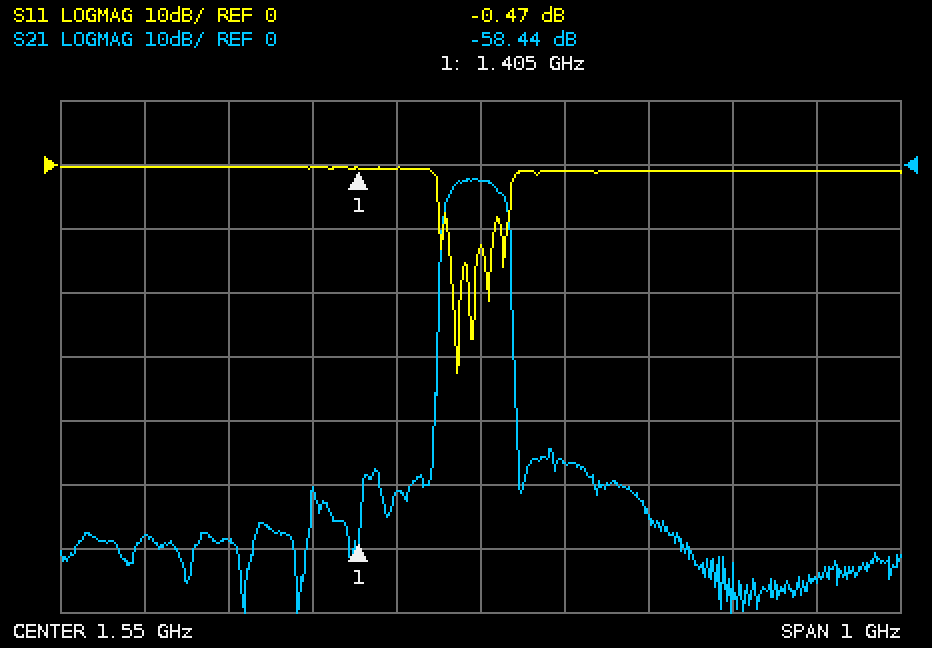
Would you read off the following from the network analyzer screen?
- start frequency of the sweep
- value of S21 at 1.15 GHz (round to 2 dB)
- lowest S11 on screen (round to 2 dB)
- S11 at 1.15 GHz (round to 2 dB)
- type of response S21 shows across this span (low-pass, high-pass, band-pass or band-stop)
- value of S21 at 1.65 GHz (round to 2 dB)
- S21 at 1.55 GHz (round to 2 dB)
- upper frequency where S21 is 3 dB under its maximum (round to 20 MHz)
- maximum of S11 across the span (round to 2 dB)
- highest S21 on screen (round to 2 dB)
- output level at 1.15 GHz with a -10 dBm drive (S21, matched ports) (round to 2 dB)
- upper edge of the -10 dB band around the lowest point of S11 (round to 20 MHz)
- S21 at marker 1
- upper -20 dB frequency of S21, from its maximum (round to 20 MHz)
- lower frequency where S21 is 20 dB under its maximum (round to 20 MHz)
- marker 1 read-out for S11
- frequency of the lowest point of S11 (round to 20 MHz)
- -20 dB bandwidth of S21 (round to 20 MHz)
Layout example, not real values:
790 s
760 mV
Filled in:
1.05 GHz
-58 dB
-32 dB
0 dB
band-pass
-46 dB
-2 dB
1.58 GHz
0 dB
-2 dB
-68 dBm
1.56 GHz
-58.44 dB
1.58 GHz
1.50 GHz
-0.47 dB
1.52 GHz
80 MHz
